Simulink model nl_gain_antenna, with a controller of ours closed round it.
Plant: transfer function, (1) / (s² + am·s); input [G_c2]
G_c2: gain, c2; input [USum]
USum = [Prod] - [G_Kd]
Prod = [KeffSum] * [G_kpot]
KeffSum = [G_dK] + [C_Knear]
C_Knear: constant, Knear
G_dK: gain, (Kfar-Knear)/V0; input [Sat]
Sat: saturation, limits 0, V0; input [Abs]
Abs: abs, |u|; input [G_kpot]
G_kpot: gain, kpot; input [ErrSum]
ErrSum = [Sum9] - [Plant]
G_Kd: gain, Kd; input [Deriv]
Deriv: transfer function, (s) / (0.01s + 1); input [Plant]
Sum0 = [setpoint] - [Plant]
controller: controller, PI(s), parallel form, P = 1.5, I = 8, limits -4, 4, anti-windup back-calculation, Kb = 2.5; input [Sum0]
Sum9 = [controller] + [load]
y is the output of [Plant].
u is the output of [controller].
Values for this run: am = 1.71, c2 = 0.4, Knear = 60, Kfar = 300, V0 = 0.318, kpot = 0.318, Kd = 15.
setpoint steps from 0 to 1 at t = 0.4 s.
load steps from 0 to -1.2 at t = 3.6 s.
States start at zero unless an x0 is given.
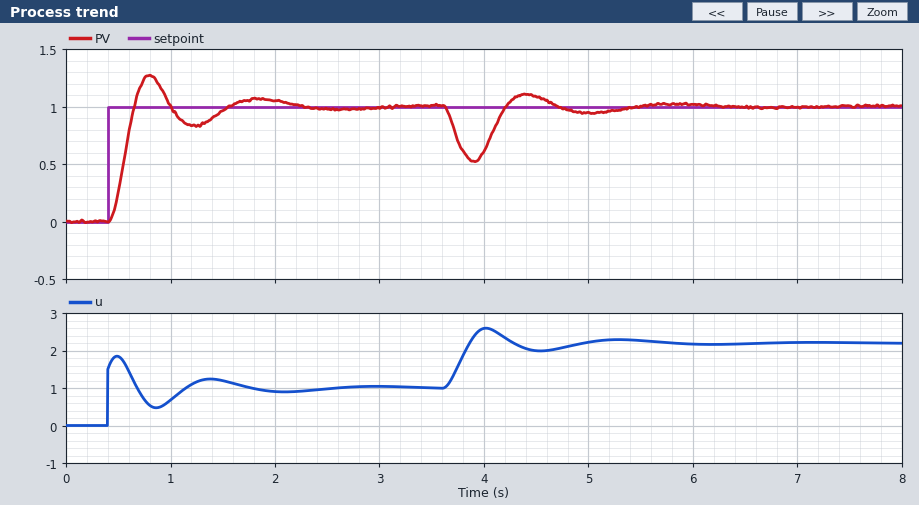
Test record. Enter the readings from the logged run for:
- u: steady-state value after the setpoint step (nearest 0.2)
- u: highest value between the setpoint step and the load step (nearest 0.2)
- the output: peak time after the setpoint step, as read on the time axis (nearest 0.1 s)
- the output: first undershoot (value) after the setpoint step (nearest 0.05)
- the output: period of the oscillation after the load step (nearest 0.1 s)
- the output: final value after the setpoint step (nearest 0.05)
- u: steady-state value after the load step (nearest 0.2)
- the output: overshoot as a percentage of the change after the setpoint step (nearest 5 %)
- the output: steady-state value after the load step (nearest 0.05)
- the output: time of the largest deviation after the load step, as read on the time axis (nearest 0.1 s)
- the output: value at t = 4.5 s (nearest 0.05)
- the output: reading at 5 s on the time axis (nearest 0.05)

1.0
1.8
0.8 s
0.85
1.1 s
1.00
2.2
25 %
1.00
3.9 s
1.10
0.95
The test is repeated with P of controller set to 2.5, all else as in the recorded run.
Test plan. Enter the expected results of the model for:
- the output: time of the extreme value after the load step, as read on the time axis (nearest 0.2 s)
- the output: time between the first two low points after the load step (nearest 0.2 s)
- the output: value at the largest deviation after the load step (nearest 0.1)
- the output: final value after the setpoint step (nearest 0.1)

3.8 s
1.0 s
0.6
1.0
